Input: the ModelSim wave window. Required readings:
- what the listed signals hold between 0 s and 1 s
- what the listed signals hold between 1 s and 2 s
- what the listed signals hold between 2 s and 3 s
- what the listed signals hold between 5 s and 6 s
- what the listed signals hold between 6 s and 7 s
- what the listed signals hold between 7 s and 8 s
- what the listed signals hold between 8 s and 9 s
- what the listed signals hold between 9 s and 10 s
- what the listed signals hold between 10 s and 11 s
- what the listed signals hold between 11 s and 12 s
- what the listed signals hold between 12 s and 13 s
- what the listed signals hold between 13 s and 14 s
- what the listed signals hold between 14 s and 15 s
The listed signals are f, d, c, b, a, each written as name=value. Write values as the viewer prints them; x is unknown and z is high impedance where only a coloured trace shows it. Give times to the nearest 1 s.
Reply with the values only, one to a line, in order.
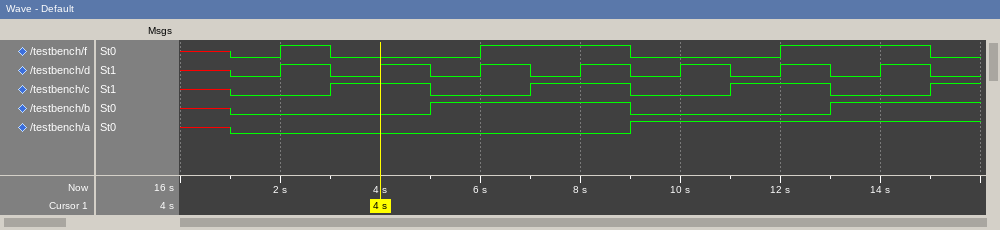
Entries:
f=x, d=x, c=x, b=x, a=x
f=0, d=0, c=0, b=0, a=0
f=1, d=1, c=0, b=0, a=0
f=0, d=0, c=0, b=1, a=0
f=1, d=1, c=0, b=1, a=0
f=1, d=0, c=1, b=1, a=0
f=1, d=1, c=1, b=1, a=0
f=0, d=0, c=0, b=0, a=1
f=0, d=1, c=0, b=0, a=1
f=0, d=0, c=1, b=0, a=1
f=1, d=1, c=1, b=0, a=1
f=1, d=0, c=0, b=1, a=1
f=1, d=1, c=0, b=1, a=1
